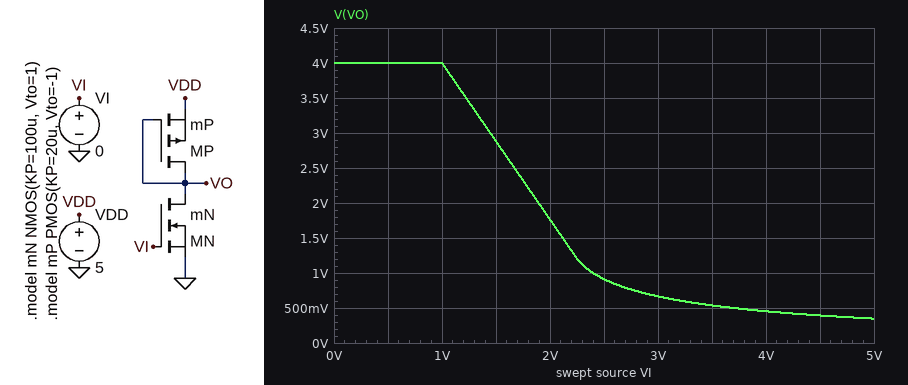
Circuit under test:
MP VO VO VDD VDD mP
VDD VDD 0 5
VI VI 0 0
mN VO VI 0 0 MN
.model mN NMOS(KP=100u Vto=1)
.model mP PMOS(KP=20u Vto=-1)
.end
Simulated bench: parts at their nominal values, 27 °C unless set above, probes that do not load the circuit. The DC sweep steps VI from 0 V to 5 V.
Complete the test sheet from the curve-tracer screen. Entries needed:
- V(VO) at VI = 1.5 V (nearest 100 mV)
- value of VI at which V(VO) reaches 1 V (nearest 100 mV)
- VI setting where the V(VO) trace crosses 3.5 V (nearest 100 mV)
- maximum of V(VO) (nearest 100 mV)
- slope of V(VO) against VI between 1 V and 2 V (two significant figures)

2.9 V
2.4 V
1.2 V
4.0 V
-2.2 V/V
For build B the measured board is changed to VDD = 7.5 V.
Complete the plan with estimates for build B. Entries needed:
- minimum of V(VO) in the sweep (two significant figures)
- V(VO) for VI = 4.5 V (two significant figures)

890 mV
1.0 V
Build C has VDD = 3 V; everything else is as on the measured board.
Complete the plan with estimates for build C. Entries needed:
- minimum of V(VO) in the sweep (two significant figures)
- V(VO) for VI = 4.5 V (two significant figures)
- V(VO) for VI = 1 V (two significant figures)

92 mV
100 mV
2.0 V
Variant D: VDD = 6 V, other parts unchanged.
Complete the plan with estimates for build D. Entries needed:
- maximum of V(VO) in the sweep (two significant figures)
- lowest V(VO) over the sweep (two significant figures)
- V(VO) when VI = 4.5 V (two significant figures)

5.0 V
530 mV
600 mV
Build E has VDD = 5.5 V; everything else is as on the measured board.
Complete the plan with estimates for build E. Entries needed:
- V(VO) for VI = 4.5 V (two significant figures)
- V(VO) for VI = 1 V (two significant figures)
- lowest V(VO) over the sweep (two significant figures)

490 mV
4.5 V
440 mV
